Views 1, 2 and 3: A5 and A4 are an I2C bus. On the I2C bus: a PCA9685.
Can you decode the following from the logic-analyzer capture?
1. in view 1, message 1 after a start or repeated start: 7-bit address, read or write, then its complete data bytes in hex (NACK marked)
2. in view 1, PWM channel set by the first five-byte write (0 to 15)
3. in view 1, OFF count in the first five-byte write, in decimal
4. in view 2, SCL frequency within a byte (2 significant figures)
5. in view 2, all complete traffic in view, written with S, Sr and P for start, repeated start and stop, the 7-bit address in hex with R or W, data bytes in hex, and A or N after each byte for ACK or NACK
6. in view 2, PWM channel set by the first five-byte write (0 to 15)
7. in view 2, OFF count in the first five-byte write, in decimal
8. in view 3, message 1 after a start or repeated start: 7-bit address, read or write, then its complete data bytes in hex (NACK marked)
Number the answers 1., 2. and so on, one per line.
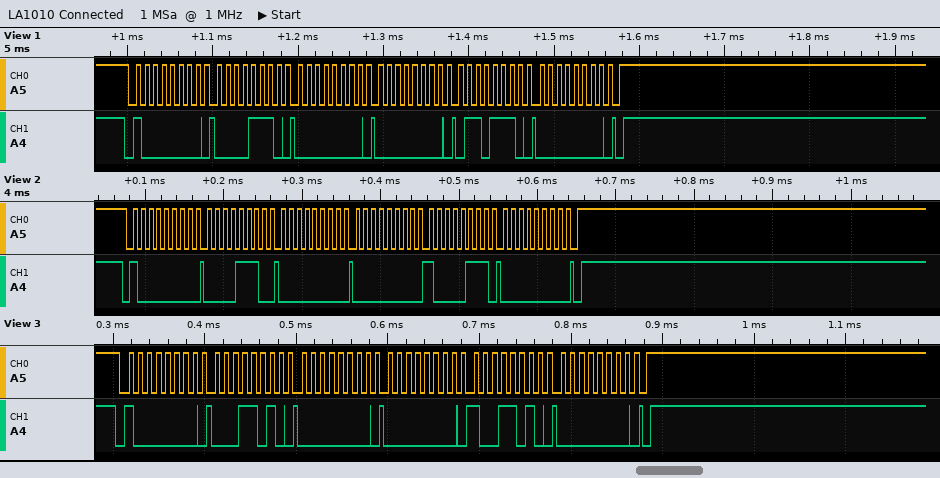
1. 0x40 write: 0E 00 00 6E 00
2. 2
3. 110
4. 100 kHz
5. S 40W A 0E A 00 A 00 A 87 A 00 A P
6. 2
7. 135
8. 0x40 write: 1A 00 00 9A 00
